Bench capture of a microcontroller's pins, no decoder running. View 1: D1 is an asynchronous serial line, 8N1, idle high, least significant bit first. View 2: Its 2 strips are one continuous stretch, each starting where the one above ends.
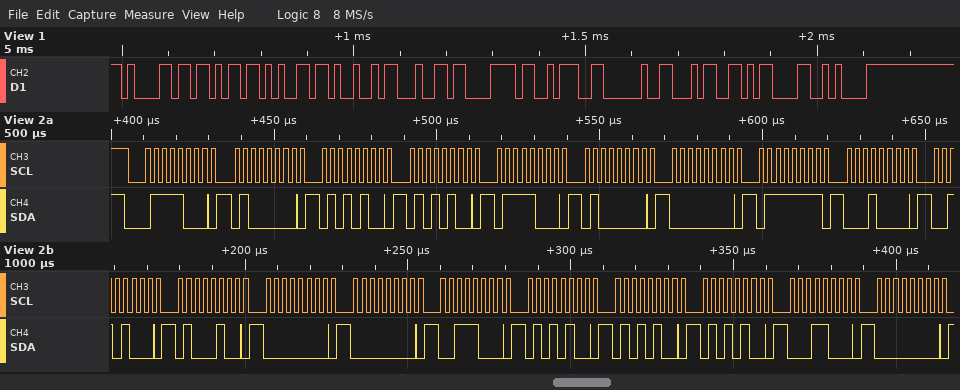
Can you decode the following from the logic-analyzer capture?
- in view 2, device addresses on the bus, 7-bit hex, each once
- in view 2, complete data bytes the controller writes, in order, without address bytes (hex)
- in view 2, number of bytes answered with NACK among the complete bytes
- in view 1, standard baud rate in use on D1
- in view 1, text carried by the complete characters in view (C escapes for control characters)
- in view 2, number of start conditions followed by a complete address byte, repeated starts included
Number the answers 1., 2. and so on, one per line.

1. 0x3C
2. 40 54 54 78 40 00 7F 10 28 44 00 00 38 54 54 54 18 00
3. 0
4. 74880 baud
5. "akeIdx: 4\r\n"
6. 1
